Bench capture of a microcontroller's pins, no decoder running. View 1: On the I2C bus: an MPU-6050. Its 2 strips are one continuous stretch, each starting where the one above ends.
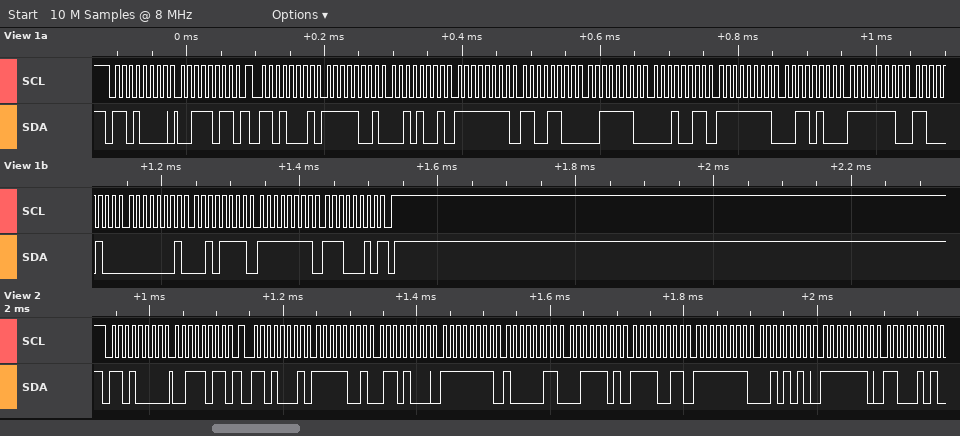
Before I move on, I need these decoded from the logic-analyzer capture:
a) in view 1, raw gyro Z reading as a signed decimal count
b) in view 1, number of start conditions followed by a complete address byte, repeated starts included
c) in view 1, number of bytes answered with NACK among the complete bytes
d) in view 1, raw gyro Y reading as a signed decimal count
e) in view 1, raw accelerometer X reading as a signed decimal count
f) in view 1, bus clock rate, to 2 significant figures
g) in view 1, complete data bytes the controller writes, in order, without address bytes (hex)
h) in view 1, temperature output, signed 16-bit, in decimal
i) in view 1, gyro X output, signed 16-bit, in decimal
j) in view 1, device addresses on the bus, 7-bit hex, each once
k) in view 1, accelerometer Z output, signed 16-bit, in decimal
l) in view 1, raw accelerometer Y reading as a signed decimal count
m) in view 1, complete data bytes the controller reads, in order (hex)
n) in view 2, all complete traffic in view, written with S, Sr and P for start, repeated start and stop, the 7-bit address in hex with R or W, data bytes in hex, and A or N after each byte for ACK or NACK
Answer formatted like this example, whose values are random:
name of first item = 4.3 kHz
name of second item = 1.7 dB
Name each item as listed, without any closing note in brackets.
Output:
in view 1, raw gyro Z reading as a signed decimal count = -30
in view 1, number of start conditions followed by a complete address byte, repeated starts included = 2
in view 1, number of bytes answered with NACK among the complete bytes = 1
in view 1, raw gyro Y reading as a signed decimal count = 303
in view 1, raw accelerometer X reading as a signed decimal count = -1751
in view 1, bus clock rate, to 2 significant figures = 100 kHz
in view 1, complete data bytes the controller writes, in order, without address bytes = 3B
in view 1, temperature output, signed 16-bit, in decimal = -204
in view 1, gyro X output, signed 16-bit, in decimal = -316
in view 1, device addresses on the bus, 7-bit hex, each once = 0x68
in view 1, accelerometer Z output, signed 16-bit, in decimal = 15891
in view 1, raw accelerometer Y reading as a signed decimal count = -52
in view 1, complete data bytes the controller reads, in order = F9 29 FF CC 3E 13 FF 34 FE C4 01 2F FF E2
in view 2, all complete traffic in view, written with S, Sr and P for start, repeated start and stop, the 7-bit address in hex with R or W, data bytes in hex, and A or N after each byte for ACK or NACK = S 68W A 3B A Sr 68R A F9 A 68 A FF A 83 A 3D A F3 A FF A 2A A FE A C5 A
